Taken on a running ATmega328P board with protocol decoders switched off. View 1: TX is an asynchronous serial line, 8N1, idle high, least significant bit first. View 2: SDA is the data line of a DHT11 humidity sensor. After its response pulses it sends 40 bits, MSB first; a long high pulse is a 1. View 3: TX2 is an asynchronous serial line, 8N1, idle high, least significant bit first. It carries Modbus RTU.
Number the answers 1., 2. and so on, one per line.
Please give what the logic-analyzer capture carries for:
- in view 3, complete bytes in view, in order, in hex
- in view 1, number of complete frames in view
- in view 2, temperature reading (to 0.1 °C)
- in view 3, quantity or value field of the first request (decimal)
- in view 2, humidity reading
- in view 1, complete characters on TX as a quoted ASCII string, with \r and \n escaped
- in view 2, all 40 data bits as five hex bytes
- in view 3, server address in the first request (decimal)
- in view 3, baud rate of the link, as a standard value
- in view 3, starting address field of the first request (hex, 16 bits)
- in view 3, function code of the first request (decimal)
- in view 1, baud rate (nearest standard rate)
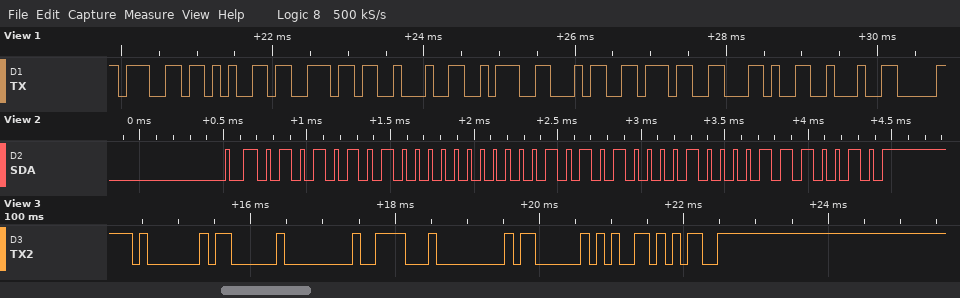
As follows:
1. 01 03 00 1E 00 03 65 CD
2. 9
3. 21.8 °C
4. 3
5. 85 %
6. "gen\":47,\""
7. 55 00 15 08 72
8. 1
9. 9600 baud
10. 0x001E
11. 3
12. 9600 baud
